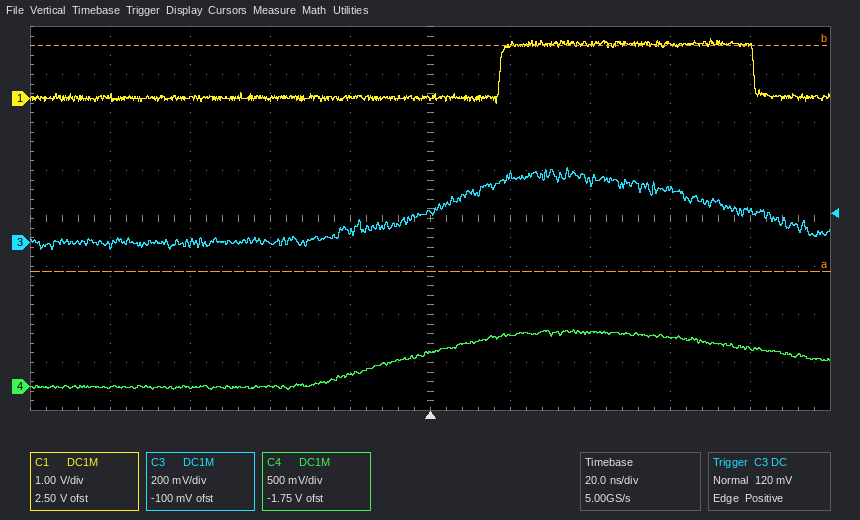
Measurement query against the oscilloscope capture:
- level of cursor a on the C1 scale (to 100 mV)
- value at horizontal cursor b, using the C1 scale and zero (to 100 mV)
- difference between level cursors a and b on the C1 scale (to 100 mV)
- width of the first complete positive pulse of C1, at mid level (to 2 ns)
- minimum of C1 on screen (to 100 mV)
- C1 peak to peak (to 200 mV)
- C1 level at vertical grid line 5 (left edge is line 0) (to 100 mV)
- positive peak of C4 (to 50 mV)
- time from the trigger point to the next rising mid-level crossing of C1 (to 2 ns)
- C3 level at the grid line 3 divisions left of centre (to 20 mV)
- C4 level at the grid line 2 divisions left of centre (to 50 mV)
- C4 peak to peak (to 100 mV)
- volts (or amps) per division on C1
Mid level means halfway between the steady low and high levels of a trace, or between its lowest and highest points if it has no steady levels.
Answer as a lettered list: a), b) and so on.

a) -3.6 V
b) 1.1 V
c) 4.7 V
d) 64 ns
e) -100 mV
f) 1.4 V
g) 0.0 V
h) 600 mV
i) 18 ns
j) 0 mV
k) 0 mV
l) 600 mV
m) 1 V
